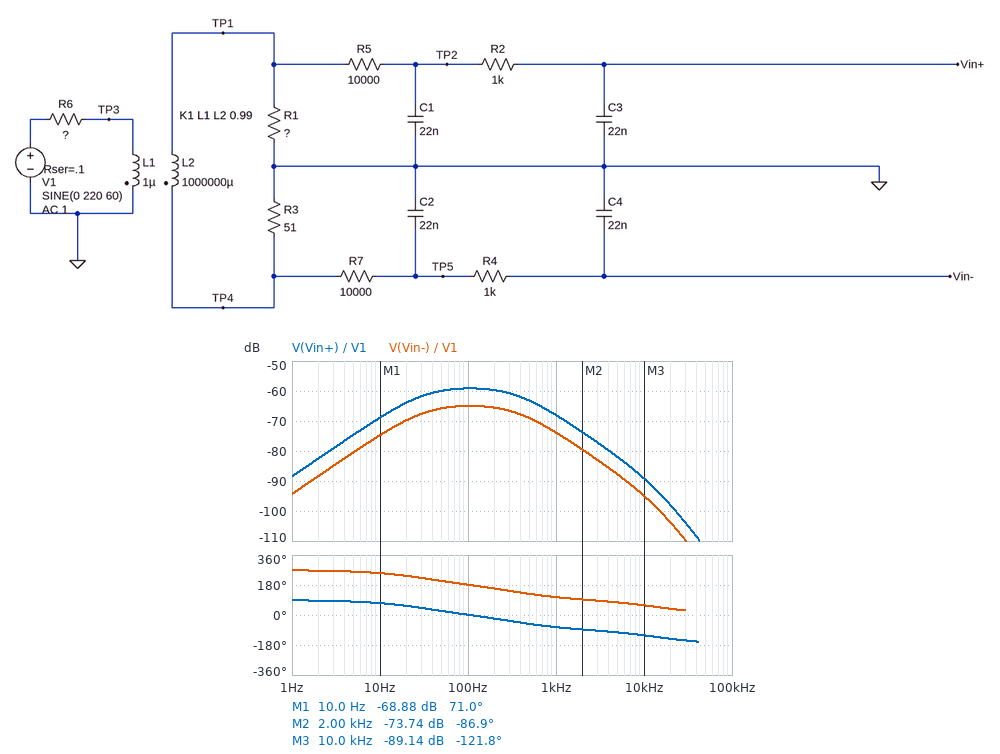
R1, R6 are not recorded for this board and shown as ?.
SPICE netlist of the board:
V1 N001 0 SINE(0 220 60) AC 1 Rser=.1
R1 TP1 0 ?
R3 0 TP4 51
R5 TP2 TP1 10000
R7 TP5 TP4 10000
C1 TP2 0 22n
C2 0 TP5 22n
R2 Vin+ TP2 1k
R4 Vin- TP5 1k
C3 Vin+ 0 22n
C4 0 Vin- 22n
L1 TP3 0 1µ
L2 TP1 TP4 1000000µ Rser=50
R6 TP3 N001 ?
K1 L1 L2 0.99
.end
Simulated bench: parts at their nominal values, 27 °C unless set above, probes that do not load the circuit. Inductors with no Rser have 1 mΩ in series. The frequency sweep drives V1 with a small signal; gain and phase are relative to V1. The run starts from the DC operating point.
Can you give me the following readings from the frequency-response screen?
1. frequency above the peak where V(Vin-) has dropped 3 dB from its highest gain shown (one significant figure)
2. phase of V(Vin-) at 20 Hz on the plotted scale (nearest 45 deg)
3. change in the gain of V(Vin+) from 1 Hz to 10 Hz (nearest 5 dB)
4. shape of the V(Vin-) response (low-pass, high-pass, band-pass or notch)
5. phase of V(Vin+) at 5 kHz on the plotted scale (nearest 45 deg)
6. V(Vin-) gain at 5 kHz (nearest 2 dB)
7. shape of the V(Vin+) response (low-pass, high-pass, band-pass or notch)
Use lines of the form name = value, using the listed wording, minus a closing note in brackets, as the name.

frequency above the peak where V(Vin-) has dropped 3 dB from its highest gain shown = 400 Hz
phase of V(Vin-) at 20 Hz on the plotted scale = 225 deg
change in the gain of V(Vin+) from 1 Hz to 10 Hz = 20 dB
shape of the V(Vin-) response = band-pass
phase of V(Vin+) at 5 kHz on the plotted scale = -90 deg
V(Vin-) gain at 5 kHz = -88 dB
shape of the V(Vin+) response = band-pass
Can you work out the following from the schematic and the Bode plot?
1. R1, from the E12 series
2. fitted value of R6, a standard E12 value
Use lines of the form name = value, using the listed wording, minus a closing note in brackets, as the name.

R1, from the E12 series = 100 Ω
fitted value of R6, a standard E12 value = 82 Ω
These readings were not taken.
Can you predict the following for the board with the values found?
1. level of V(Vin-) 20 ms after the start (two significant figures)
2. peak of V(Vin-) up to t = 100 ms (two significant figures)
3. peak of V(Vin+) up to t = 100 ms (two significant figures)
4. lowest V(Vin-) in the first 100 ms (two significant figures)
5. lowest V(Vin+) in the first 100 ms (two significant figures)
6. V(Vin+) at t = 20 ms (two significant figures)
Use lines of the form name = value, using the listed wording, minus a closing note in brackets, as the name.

level of V(Vin-) 20 ms after the start = -120 mV
peak of V(Vin-) up to t = 100 ms = 120 mV
peak of V(Vin+) up to t = 100 ms = 230 mV
lowest V(Vin-) in the first 100 ms = -120 mV
lowest V(Vin+) in the first 100 ms = -240 mV
V(Vin+) at t = 20 ms = 230 mV
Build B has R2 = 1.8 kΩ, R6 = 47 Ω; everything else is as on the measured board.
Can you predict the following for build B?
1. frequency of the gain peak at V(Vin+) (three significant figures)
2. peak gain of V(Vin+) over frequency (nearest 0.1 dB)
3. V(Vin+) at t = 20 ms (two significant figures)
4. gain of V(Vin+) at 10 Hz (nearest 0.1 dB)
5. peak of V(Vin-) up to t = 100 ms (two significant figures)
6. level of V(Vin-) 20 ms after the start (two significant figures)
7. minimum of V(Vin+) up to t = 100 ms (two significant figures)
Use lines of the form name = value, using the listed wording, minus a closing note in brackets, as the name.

frequency of the gain peak at V(Vin+) = 105 Hz
peak gain of V(Vin+) over frequency = -54.3 dB
V(Vin+) at t = 20 ms = 400 mV
gain of V(Vin+) at 10 Hz = -64.1 dB
peak of V(Vin-) up to t = 100 ms = 220 mV
level of V(Vin-) 20 ms after the start = -200 mV
minimum of V(Vin+) up to t = 100 ms = -420 mV
